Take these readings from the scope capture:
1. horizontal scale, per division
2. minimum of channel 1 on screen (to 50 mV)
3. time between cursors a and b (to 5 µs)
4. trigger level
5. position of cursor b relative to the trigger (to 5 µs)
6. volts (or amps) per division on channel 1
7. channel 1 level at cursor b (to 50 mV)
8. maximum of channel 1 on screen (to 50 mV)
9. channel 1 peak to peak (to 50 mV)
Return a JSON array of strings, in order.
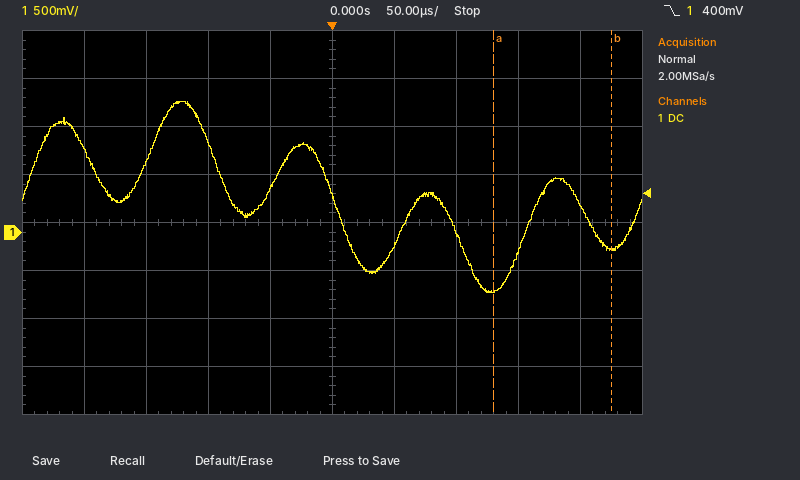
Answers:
["50 µs", "-650 mV", "95 µs", "400 mV", "+225 µs", "500 mV", "-200 mV", "1.35 V", "2.00 V"]
